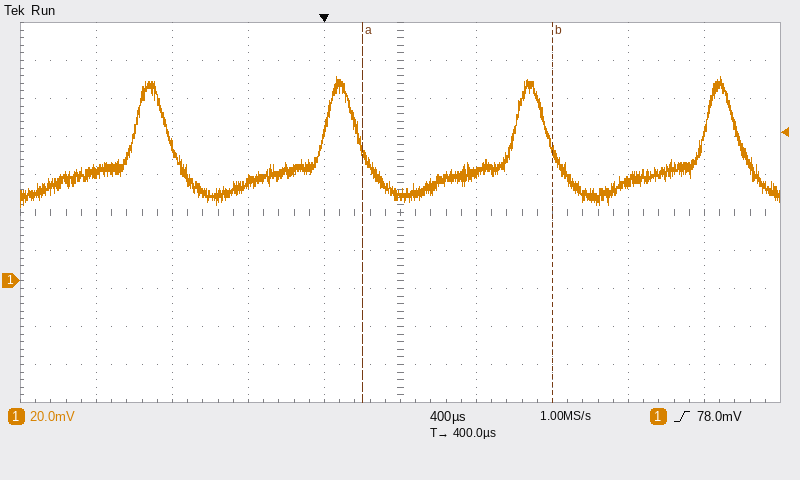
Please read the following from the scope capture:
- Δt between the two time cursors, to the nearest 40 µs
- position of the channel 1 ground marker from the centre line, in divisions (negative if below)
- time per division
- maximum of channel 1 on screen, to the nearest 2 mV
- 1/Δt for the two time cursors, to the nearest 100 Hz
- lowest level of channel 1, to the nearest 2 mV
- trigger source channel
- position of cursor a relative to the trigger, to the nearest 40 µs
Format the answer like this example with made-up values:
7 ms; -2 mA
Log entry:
1.00 ms; -1.8 div; 400 µs; 108 mV; 1.0 kHz; 38 mV; channel 1; +200 µs
